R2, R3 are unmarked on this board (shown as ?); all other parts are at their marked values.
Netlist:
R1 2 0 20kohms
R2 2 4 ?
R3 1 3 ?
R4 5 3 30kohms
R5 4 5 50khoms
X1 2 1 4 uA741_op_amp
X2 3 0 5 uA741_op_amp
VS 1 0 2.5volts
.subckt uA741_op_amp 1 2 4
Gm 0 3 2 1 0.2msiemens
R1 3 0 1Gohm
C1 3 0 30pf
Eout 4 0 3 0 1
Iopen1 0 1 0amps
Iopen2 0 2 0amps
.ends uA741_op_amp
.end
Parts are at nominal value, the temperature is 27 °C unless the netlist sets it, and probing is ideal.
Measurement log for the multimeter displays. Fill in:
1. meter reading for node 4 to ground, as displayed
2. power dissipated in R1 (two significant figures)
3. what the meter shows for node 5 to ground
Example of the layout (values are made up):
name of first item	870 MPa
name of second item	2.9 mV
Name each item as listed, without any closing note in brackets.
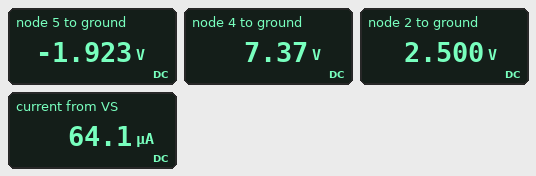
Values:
meter reading for node 4 to ground, as displayed	7.37 V
power dissipated in R1	310 µW
what the meter shows for node 5 to ground	-1.923 V
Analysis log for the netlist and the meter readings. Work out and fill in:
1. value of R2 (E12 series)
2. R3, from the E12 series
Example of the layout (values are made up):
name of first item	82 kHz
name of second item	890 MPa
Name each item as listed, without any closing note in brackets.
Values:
value of R2	39 kΩ
R3, from the E12 series	39 kΩ
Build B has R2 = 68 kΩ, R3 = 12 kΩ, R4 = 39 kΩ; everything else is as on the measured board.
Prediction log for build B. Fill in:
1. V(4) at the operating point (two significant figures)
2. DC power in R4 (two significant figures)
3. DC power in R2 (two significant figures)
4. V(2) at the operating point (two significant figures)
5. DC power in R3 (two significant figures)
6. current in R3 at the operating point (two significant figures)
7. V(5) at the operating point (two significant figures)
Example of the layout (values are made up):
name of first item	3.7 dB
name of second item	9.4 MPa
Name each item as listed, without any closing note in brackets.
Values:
V(4) at the operating point	11 V
DC power in R4	1.7 mW
DC power in R2	1.1 mW
V(2) at the operating point	2.5 V
DC power in R3	520 µW
current in R3 at the operating point	210 µA
V(5) at the operating point	-8.1 V
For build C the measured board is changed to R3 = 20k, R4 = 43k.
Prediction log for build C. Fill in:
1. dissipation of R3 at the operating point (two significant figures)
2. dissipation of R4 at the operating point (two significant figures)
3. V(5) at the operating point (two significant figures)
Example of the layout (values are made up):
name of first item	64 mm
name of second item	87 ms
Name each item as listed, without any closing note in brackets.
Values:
dissipation of R3 at the operating point	310 µW
dissipation of R4 at the operating point	670 µW
V(5) at the operating point	-5.4 V
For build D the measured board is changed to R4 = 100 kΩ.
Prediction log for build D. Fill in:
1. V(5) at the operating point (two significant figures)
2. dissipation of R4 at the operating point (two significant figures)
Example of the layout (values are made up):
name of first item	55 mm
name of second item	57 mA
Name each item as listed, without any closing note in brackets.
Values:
V(5) at the operating point	-6.4 V
dissipation of R4 at the operating point	410 µW
